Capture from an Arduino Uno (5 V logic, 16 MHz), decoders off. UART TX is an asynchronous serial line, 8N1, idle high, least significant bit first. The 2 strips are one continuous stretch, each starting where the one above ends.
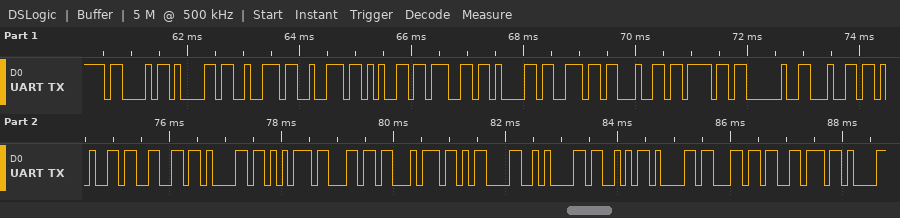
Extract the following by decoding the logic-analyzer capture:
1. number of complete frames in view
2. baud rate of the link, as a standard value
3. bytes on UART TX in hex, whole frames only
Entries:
24
9600 baud
43 61 72 72 65 67 61 6E 64 6F 20 64 65 66 61 75 6C 74 0D 0A 53 61 6C 76
